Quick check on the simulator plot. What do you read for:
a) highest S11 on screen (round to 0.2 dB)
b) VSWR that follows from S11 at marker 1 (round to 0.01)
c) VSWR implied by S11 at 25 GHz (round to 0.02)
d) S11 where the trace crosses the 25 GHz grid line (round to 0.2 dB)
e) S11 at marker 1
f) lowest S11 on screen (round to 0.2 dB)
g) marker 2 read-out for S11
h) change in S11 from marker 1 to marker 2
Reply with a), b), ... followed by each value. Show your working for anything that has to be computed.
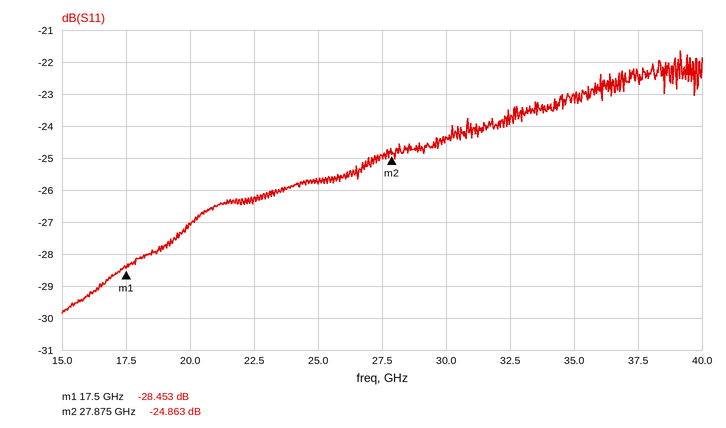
a) -21.6 dB
b) (1 + 0.0378)/(1 − 0.0378) ≈ 1.08
c) |Γ| = 10^(-25.8/20) = 0.0513; VSWR = (1 + 0.0513)/(1 − 0.0513) ≈ 1.11, so 1.10 to the nearest 0.02
d) -25.8 dB
e) -28.453 dB
f) -29.8 dB
g) -24.863 dB
h) -24.863 − (-28.453) = 3.590 dB
